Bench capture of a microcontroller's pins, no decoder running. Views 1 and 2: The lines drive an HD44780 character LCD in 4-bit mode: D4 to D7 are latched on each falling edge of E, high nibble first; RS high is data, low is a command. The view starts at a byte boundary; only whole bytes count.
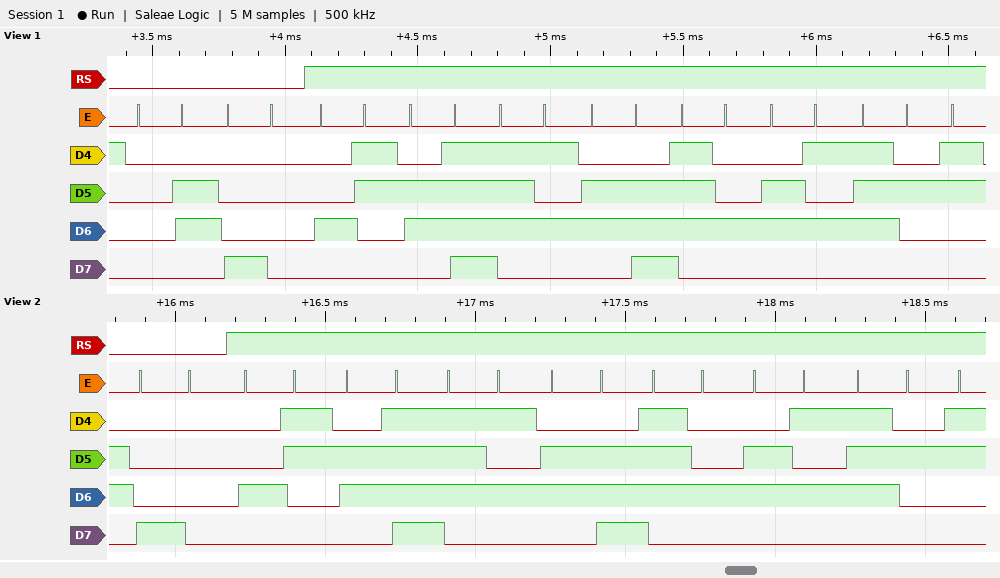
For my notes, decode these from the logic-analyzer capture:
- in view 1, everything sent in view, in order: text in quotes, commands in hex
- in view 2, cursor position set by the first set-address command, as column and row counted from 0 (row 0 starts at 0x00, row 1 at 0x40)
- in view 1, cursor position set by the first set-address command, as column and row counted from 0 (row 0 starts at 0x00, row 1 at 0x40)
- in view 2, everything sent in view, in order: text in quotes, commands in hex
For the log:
0x06 0x80 "Counter"
column 0, row 0
column 0, row 0
0x80 "Counter"
